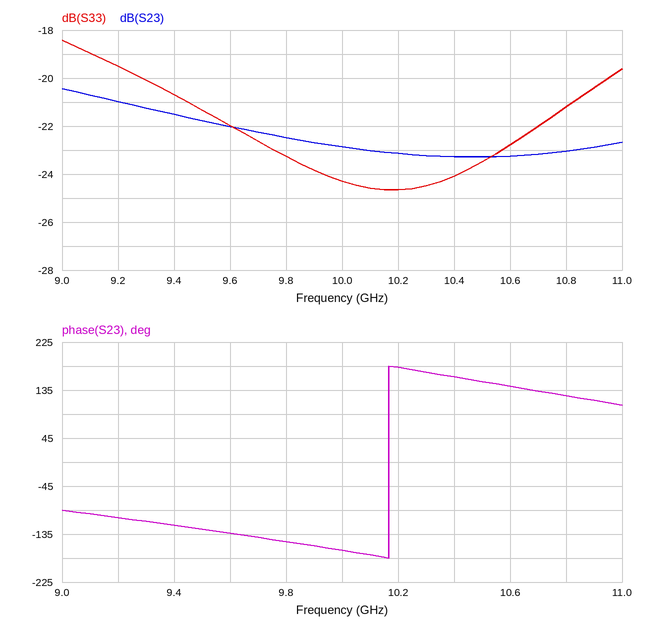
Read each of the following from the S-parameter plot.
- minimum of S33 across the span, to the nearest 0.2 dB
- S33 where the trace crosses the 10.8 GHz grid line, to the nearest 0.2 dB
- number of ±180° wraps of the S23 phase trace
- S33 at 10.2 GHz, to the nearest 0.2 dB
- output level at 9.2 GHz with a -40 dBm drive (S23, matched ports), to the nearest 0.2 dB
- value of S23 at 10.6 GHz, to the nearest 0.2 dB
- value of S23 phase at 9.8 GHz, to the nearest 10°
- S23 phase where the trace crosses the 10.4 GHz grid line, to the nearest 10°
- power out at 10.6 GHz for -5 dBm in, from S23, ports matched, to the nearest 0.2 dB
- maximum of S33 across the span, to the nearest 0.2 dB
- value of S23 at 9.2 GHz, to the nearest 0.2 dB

-24.6 dB
-21.2 dB
1
-24.6 dB
-61.0 dBm
-23.2 dB
-150°
160°
-28.2 dBm
-18.4 dB
-21.0 dB
